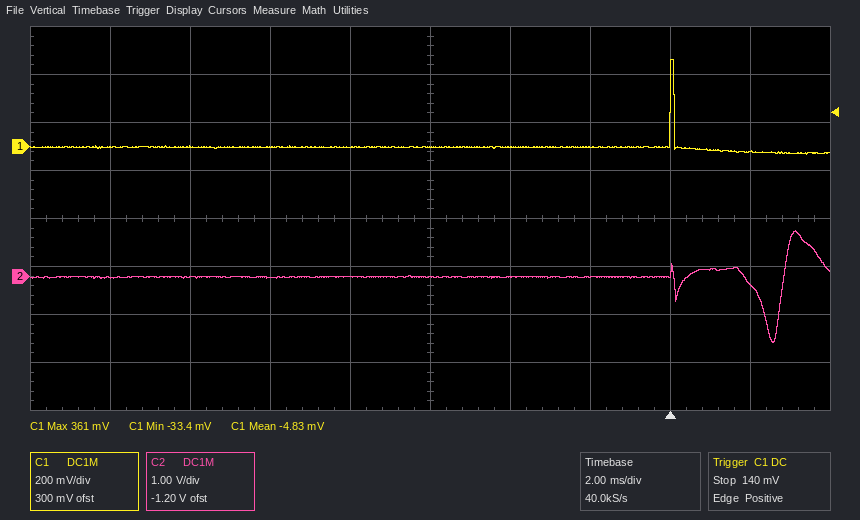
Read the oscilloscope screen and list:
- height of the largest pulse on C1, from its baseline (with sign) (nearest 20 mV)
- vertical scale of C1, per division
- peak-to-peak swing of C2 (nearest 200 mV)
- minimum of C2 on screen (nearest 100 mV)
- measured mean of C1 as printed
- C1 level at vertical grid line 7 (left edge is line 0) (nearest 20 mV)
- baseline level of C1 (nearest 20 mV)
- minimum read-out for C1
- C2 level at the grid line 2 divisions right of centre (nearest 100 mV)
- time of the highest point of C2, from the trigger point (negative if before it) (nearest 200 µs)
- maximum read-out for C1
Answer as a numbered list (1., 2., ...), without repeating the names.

1. +360 mV
2. 200 mV
3. 2.4 V
4. -1.4 V
5. -4.83 mV
6. 0 mV
7. 0 mV
8. -33.4 mV
9. 0.0 V
10. +3.2 ms
11. 361 mV
